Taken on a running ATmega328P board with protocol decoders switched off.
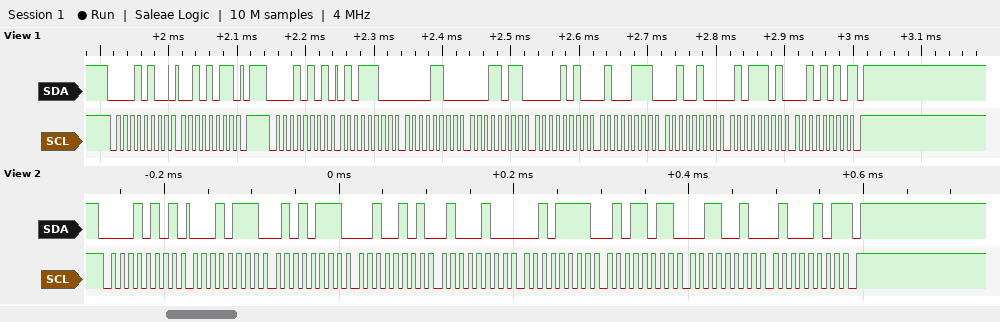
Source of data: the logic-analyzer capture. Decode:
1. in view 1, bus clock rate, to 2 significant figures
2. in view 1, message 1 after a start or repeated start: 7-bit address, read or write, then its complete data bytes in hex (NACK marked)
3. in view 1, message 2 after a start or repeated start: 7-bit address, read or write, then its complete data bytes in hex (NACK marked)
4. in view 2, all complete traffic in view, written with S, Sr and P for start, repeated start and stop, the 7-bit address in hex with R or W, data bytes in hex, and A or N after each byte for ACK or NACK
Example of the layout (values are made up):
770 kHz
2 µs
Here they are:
100 kHz
0x0A write: 2B
0x0A read: 5C 0C 1B 0A 47 24 5D 2A NACK
S 0AR A 17 A 57 A 25 A 44 A 2F A 5B A 32 A 45 N P
